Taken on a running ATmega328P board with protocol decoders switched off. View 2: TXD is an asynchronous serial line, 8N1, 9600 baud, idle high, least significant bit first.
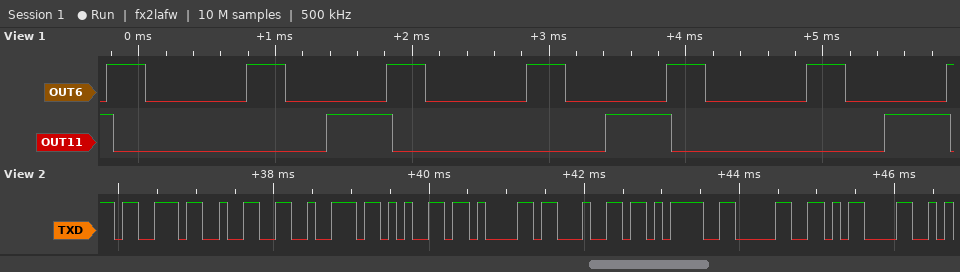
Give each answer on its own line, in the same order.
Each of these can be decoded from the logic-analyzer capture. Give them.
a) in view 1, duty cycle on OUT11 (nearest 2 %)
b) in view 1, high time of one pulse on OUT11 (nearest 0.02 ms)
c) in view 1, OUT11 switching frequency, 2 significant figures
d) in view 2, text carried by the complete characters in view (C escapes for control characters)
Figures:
24 %
0.48 ms
490 Hz
"s2read=0\r"
